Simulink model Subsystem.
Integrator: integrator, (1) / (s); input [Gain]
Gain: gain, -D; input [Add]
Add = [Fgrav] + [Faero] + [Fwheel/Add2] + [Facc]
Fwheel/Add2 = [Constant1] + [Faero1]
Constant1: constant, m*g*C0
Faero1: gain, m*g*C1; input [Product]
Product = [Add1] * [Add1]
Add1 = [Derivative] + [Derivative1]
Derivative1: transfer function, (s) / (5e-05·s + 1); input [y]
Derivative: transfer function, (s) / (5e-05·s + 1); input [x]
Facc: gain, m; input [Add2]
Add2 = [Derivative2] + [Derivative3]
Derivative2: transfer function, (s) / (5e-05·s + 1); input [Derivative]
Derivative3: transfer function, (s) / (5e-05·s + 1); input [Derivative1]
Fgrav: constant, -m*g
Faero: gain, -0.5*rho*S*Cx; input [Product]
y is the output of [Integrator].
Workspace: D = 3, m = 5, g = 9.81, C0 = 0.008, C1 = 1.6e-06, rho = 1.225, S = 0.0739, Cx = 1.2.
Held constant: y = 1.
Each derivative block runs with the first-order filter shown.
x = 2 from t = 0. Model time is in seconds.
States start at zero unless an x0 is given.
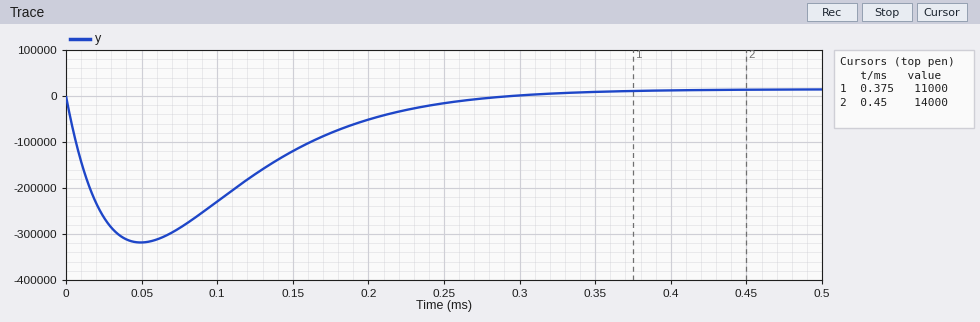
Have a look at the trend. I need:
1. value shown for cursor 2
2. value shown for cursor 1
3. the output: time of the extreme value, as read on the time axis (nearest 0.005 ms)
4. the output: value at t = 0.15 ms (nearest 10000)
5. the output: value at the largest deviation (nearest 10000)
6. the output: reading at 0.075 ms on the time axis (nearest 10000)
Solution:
14000
11000
0.050 ms
-120000
-320000
-290000
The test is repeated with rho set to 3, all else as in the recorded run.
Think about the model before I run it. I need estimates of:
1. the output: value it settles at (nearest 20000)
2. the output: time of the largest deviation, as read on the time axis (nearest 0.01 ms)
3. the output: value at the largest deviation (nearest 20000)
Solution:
40000
0.05 ms
-300000
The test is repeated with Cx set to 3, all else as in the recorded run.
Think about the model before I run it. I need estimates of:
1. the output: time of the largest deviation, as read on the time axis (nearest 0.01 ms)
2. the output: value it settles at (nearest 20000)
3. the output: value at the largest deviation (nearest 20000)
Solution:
0.05 ms
40000
-300000
